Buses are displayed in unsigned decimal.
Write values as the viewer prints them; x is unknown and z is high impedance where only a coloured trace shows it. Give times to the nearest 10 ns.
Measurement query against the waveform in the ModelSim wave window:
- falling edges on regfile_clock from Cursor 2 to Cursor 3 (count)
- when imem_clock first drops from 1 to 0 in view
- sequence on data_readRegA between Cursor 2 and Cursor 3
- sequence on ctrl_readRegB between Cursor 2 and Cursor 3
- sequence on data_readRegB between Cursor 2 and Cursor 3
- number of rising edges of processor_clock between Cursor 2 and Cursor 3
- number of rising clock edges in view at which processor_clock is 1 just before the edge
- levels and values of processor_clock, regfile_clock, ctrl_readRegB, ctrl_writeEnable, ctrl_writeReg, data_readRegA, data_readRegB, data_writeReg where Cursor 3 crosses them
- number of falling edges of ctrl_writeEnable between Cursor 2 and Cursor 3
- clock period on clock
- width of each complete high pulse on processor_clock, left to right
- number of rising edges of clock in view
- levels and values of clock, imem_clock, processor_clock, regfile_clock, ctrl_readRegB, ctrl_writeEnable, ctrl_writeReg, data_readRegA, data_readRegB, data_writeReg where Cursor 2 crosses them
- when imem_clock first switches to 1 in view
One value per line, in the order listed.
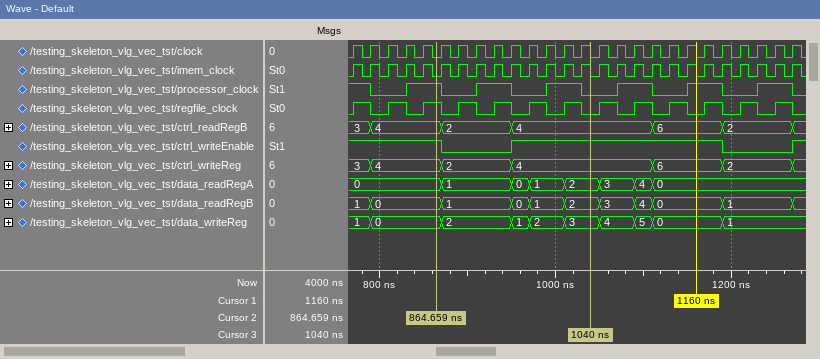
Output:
5
780 ns
0, 1, 0, 1, 2
4, 2, 4
0, 1, 0, 1, 2
2
14
processor_clock=0, regfile_clock=0, ctrl_readRegB=4, ctrl_writeEnable=1, ctrl_writeReg=4, data_readRegA=2, data_readRegB=2, data_writeReg=3
1
20 ns
40 ns, 40 ns, 40 ns, 40 ns, 40 ns, 40 ns
26
clock=0, imem_clock=0, processor_clock=1, regfile_clock=1, ctrl_readRegB=4, ctrl_writeEnable=1, ctrl_writeReg=4, data_readRegA=0, data_readRegB=0, data_writeReg=0
770 ns
